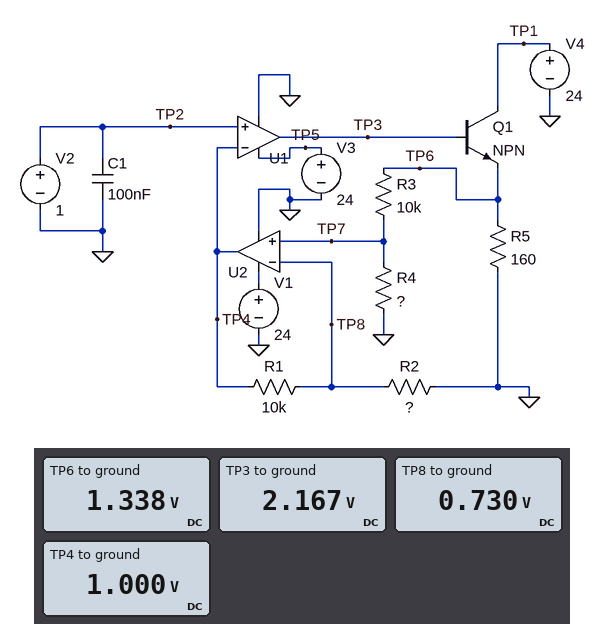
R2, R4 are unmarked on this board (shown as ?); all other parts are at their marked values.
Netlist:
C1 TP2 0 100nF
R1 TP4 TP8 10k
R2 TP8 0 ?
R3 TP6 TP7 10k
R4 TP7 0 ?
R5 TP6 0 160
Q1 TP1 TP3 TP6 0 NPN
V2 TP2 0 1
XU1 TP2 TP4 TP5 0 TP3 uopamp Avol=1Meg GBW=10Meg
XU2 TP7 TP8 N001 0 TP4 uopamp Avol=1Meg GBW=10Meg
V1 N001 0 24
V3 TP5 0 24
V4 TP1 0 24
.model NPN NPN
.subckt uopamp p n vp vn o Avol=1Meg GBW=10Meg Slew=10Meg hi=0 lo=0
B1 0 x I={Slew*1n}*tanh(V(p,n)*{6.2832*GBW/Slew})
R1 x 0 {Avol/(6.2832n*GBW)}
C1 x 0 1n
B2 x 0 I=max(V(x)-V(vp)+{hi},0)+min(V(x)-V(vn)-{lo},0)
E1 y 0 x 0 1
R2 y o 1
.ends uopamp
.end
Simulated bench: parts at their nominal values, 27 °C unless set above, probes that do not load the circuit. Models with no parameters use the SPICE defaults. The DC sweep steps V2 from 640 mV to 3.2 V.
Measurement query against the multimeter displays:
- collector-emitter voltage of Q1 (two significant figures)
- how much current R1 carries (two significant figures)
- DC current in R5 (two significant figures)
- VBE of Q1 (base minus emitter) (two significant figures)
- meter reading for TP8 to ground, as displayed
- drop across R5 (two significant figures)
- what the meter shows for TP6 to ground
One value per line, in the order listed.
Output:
23 V
27 µA
8.4 mA
830 mV
0.730 V
1.3 V
1.338 V
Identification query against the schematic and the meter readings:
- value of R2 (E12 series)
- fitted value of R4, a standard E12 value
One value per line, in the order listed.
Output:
27 kΩ
12 kΩ
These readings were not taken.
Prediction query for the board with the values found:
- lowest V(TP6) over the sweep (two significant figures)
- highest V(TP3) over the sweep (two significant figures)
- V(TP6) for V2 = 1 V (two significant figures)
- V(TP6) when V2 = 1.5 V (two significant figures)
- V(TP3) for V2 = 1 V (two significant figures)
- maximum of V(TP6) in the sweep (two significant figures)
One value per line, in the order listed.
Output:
860 mV
5.1 V
1.3 V
2.0 V
2.2 V
4.3 V
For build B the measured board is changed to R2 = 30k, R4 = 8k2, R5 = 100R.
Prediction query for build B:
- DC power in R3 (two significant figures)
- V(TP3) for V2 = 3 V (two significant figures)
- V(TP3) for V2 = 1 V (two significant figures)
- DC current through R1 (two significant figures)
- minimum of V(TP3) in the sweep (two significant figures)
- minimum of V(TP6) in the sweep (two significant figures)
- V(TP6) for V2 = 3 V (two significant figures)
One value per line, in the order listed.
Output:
84 µW
5.9 V
2.5 V
25 µA
1.9 V
1.1 V
5.0 V
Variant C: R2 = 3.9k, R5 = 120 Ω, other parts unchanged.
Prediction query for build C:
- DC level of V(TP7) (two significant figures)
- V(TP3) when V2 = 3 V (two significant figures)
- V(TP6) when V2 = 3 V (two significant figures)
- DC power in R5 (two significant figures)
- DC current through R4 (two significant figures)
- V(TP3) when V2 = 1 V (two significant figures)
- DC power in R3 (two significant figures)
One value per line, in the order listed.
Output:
280 mV
2.4 V
1.5 V
2.2 mW
23 µA
1.3 V
5.5 µW
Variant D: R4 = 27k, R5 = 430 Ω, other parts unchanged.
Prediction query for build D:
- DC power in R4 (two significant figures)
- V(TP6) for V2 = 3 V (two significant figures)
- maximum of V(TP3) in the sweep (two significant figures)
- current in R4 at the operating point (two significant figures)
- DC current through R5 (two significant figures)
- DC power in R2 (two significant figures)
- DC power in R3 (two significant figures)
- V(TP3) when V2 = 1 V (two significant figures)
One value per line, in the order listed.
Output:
20 µW
3.0 V
4.0 V
27 µA
2.3 mA
20 µW
7.3 µW
1.8 V
